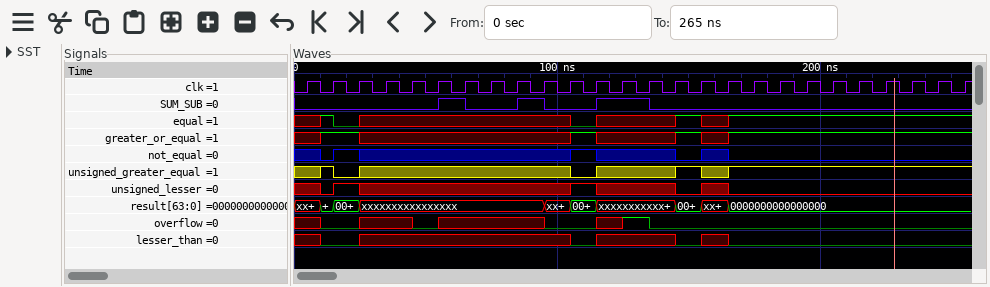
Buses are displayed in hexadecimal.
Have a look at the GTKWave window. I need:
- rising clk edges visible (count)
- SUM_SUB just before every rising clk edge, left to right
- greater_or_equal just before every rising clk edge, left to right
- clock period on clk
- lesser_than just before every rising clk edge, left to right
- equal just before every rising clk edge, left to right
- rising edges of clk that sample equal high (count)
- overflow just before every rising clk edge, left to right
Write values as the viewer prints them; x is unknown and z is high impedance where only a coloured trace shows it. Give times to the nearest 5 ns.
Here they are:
26
0 0 0 0 0 0 1 0 0 1 0 0 1 1 0 0 0 0 0 0 0 0 0 0 0 0
x 1 1 x x x x x x x x 1 x x x 1 x 1 1 1 1 1 1 1 1 1
10 ns
x 0 0 x x x x x x x x 0 x x x 0 x 0 0 0 0 0 0 0 0 0
x 1 0 x x x x x x x x 0 x x x 1 x 1 1 1 1 1 1 1 1 1
11
x 0 0 x x 0 x x x x 0 0 x 1 0 0 0 0 0 0 0 0 0 0 0 0
